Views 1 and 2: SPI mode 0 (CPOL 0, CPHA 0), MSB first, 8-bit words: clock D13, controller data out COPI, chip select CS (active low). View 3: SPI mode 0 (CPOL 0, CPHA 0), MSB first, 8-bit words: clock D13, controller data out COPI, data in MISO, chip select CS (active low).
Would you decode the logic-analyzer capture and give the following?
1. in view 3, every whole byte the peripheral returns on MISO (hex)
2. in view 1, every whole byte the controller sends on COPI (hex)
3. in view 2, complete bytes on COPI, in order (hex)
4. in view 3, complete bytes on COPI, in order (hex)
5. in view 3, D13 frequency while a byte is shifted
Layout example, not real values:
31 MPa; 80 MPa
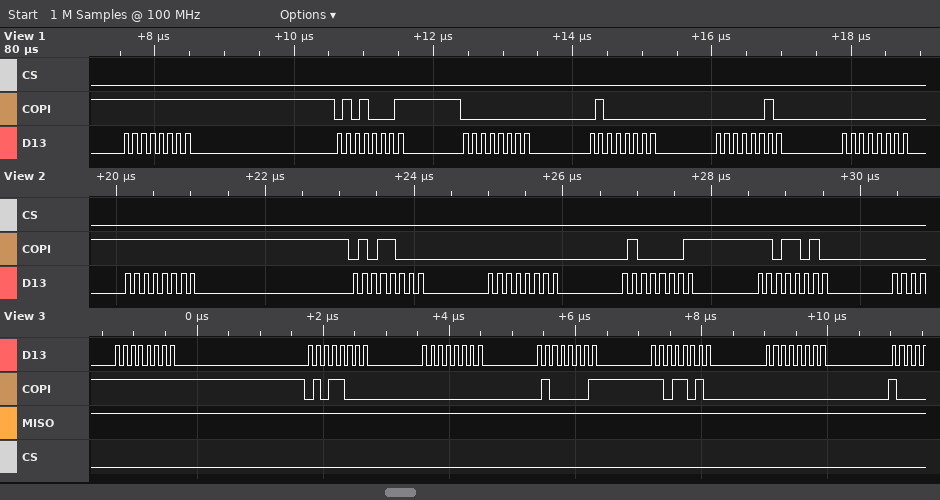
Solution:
FF FF FF FF FF FF; FF 51 00 40 02 00; FF 58 00 41 DA; FF 58 00 41 DA 00; 8 MHz
